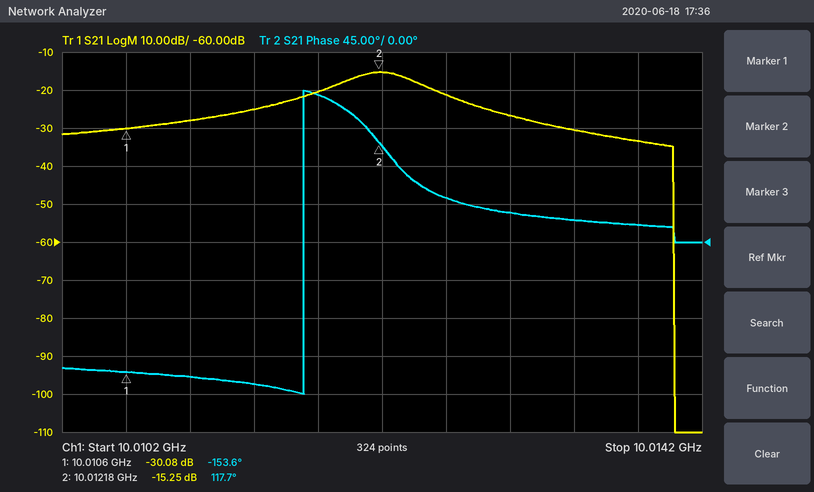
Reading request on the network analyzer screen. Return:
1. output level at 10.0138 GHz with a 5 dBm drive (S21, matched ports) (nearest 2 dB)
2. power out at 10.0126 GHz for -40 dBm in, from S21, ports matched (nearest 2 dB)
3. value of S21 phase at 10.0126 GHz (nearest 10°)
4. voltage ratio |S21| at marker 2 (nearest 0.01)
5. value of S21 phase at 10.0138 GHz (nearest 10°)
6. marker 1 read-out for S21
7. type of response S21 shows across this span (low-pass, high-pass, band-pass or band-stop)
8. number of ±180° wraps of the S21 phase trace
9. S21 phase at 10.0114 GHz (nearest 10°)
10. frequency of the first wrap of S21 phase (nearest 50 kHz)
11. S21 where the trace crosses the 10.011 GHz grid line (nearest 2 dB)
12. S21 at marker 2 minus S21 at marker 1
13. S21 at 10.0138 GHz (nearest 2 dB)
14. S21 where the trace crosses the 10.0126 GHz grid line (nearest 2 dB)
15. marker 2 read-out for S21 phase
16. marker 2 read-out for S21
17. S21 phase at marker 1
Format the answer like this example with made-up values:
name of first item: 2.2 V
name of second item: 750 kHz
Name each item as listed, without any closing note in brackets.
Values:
output level at 10.0138 GHz with a 5 dBm drive (S21, matched ports): -28 dBm
power out at 10.0126 GHz for -40 dBm in, from S21, ports matched: -62 dBm
value of S21 phase at 10.0126 GHz: 50°
voltage ratio |S21| at marker 2: 0.17
value of S21 phase at 10.0138 GHz: 20°
marker 1 read-out for S21: -30.08 dB
type of response S21 shows across this span: band-pass
number of ±180° wraps of the S21 phase trace: 1
S21 phase at 10.0114 GHz: -170°
frequency of the first wrap of S21 phase: 10.01170 GHz
S21 where the trace crosses the 10.011 GHz grid line: -28 dB
S21 at marker 2 minus S21 at marker 1: 14.83 dB
S21 at 10.0138 GHz: -34 dB
S21 where the trace crosses the 10.0126 GHz grid line: -22 dB
marker 2 read-out for S21 phase: 117.7°
marker 2 read-out for S21: -15.25 dB
S21 phase at marker 1: -153.6°
